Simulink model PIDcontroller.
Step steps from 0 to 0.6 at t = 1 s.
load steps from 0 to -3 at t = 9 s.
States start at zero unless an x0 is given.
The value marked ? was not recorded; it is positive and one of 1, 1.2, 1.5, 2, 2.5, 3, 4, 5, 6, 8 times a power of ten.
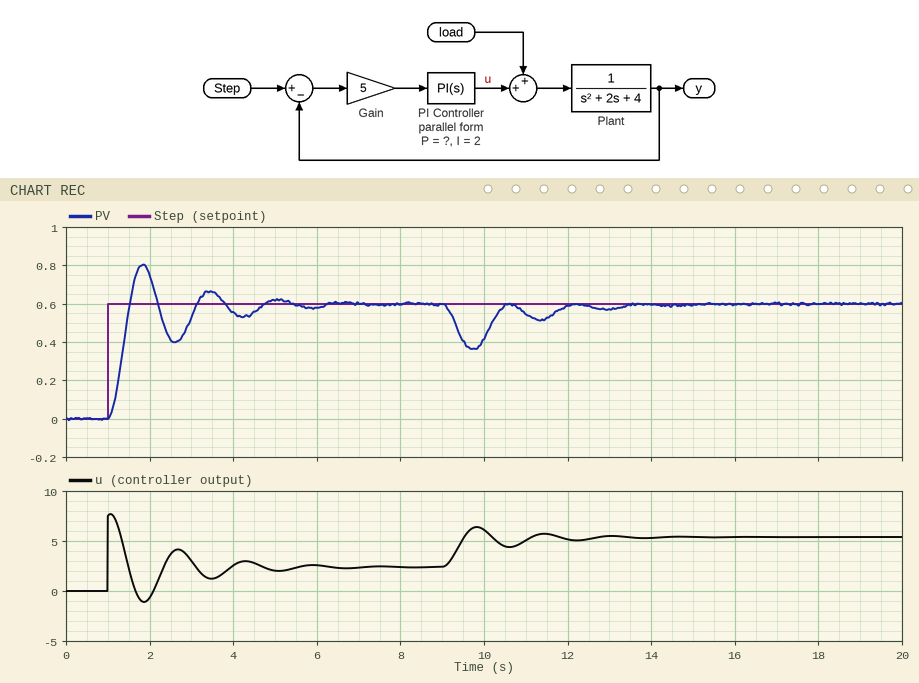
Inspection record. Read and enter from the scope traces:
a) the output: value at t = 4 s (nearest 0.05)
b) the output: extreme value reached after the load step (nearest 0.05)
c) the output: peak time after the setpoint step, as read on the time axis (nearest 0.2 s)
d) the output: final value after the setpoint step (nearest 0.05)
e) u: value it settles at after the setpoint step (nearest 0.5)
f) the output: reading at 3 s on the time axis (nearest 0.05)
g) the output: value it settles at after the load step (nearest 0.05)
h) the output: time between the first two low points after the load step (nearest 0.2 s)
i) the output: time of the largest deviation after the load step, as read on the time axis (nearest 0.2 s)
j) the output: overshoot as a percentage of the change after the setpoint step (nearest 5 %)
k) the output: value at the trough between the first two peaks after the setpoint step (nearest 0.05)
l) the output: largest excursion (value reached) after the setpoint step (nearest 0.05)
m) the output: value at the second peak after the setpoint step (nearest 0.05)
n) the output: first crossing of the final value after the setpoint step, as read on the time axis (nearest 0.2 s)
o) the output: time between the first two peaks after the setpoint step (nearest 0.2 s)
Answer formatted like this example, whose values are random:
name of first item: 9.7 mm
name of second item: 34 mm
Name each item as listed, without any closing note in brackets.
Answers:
the output: value at t = 4 s: 0.55
the output: extreme value reached after the load step: 0.35
the output: peak time after the setpoint step, as read on the time axis: 1.8 s
the output: final value after the setpoint step: 0.60
u: value it settles at after the setpoint step: 2.5
the output: reading at 3 s on the time axis: 0.55
the output: value it settles at after the load step: 0.60
the output: time between the first two low points after the load step: 1.6 s
the output: time of the largest deviation after the load step, as read on the time axis: 9.8 s
the output: overshoot as a percentage of the change after the setpoint step: 35 %
the output: value at the trough between the first two peaks after the setpoint step: 0.40
the output: largest excursion (value reached) after the setpoint step: 0.80
the output: value at the second peak after the setpoint step: 0.65
the output: first crossing of the final value after the setpoint step, as read on the time axis: 1.6 s
the output: time between the first two peaks after the setpoint step: 1.6 s
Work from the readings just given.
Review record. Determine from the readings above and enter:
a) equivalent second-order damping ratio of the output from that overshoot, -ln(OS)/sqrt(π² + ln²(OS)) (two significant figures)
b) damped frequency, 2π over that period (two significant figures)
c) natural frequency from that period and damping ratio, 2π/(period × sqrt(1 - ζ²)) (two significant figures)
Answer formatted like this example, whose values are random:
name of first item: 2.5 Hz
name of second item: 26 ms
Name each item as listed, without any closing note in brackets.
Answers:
equivalent second-order damping ratio of the output from that overshoot, -ln(OS)/sqrt(π² + ln²(OS)): 0.32
damped frequency, 2π over that period: 3.9 rad/s
natural frequency from that period and damping ratio, 2π/(period × sqrt(1 - ζ²)): 4.1 rad/s
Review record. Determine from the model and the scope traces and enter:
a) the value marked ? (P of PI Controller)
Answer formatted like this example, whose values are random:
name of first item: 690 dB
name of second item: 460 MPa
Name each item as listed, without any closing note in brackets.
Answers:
the value marked ?: 2.5
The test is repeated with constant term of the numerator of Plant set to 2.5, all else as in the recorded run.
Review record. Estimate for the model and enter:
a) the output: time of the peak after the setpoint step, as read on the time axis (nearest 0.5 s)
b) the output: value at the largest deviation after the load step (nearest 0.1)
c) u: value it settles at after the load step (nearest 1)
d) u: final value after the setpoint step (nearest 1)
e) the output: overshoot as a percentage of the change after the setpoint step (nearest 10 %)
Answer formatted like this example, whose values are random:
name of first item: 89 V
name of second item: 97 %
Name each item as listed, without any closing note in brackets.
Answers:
the output: time of the peak after the setpoint step, as read on the time axis: 1.5 s
the output: value at the largest deviation after the load step: 0.3
u: value it settles at after the load step: 4
u: final value after the setpoint step: 1
the output: overshoot as a percentage of the change after the setpoint step: 60 %
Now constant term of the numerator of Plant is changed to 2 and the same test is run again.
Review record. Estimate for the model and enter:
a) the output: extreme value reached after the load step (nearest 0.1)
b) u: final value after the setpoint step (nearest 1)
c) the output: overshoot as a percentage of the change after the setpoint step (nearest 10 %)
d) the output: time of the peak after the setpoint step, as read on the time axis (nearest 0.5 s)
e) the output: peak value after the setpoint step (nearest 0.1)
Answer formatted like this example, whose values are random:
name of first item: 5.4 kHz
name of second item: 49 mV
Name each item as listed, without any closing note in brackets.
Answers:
the output: extreme value reached after the load step: 0.3
u: final value after the setpoint step: 1
the output: overshoot as a percentage of the change after the setpoint step: 50 %
the output: time of the peak after the setpoint step, as read on the time axis: 1.5 s
the output: peak value after the setpoint step: 0.9
